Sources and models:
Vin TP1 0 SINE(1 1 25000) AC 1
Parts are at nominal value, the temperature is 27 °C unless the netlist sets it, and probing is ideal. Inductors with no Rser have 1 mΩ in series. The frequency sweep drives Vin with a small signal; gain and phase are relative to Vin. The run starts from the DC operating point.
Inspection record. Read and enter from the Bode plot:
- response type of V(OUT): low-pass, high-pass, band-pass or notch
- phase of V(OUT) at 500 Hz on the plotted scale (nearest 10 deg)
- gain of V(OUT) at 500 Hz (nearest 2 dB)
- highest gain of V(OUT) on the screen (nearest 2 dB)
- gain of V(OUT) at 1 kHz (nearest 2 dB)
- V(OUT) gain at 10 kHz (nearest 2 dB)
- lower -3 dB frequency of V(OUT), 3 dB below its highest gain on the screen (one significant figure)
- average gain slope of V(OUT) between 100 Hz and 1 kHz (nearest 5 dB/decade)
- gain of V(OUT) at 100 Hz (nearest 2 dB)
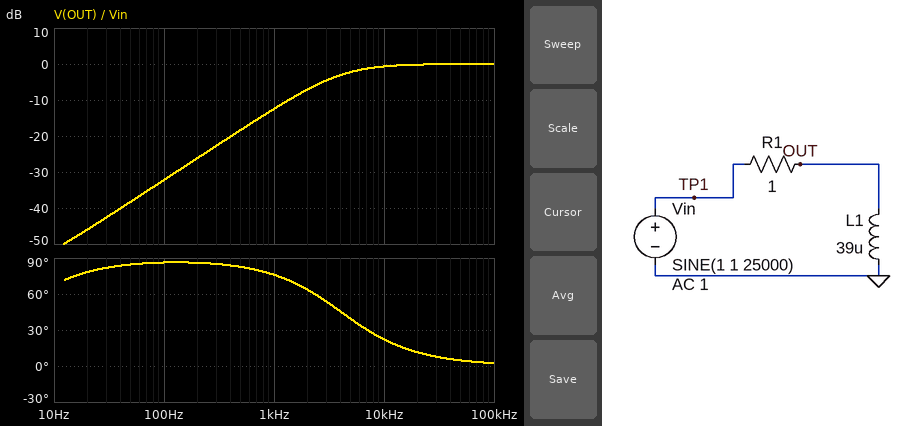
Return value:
high-pass
80 deg
-18 dB
0 dB
-12 dB
0 dB
4 kHz
20 dB/decade
-32 dB
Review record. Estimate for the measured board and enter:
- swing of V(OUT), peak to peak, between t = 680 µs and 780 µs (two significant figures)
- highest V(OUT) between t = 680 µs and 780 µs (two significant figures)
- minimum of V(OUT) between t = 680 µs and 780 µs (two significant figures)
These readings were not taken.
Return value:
2.0 V
990 mV
-990 mV
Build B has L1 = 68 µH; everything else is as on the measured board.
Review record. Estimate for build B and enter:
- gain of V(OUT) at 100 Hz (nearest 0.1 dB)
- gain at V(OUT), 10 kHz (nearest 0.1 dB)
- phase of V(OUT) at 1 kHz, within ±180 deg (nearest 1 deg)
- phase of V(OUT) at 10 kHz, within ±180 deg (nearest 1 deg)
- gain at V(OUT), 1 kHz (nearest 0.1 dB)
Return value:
-27.4 dB
-0.2 dB
67 deg
13 deg
-8.1 dB
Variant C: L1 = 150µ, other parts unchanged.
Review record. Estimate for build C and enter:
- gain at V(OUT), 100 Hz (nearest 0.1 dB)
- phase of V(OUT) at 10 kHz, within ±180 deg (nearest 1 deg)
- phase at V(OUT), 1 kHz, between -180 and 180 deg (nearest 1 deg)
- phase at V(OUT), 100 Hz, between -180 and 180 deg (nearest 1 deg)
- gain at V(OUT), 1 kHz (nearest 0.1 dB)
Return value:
-20.6 dB
6 deg
47 deg
84 deg
-3.3 dB
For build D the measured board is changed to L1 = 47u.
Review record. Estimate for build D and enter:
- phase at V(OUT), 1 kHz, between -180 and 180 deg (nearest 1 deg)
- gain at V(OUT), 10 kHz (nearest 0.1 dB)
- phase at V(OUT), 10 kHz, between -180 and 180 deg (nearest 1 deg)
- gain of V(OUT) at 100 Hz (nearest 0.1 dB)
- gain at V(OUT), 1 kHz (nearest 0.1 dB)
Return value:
73 deg
-0.5 dB
19 deg
-30.6 dB
-11.0 dB
